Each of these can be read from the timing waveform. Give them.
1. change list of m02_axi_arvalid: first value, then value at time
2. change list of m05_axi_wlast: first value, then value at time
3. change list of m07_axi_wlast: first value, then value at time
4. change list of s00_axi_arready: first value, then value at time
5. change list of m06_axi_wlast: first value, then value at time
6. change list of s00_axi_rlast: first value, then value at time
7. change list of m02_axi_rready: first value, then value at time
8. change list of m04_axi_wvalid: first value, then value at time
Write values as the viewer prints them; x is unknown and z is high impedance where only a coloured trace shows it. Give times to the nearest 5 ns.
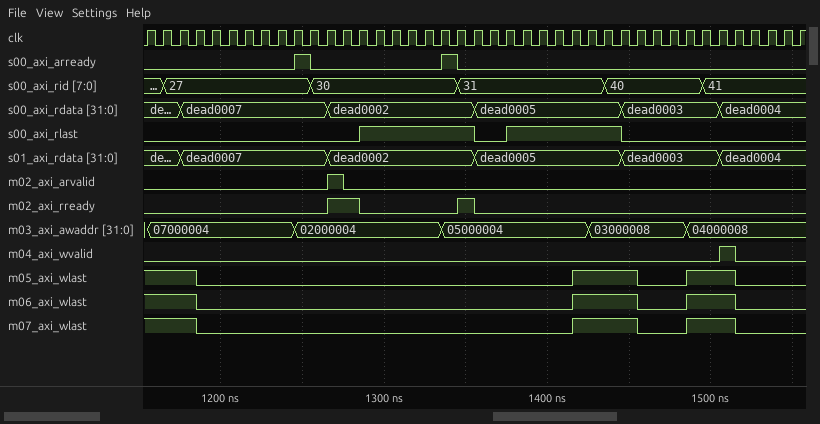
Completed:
0, 1 at 1265 ns, 0 at 1275 ns
1, 0 at 1185 ns, 1 at 1415 ns, 0 at 1455 ns, 1 at 1485 ns, 0 at 1515 ns
1, 0 at 1185 ns, 1 at 1415 ns, 0 at 1455 ns, 1 at 1485 ns, 0 at 1515 ns
0, 1 at 1245 ns, 0 at 1255 ns, 1 at 1335 ns, 0 at 1345 ns
1, 0 at 1185 ns, 1 at 1415 ns, 0 at 1455 ns, 1 at 1485 ns, 0 at 1515 ns
0, 1 at 1285 ns, 0 at 1355 ns, 1 at 1375 ns, 0 at 1445 ns
0, 1 at 1265 ns, 0 at 1285 ns, 1 at 1345 ns, 0 at 1355 ns
0, 1 at 1505 ns, 0 at 1515 ns
